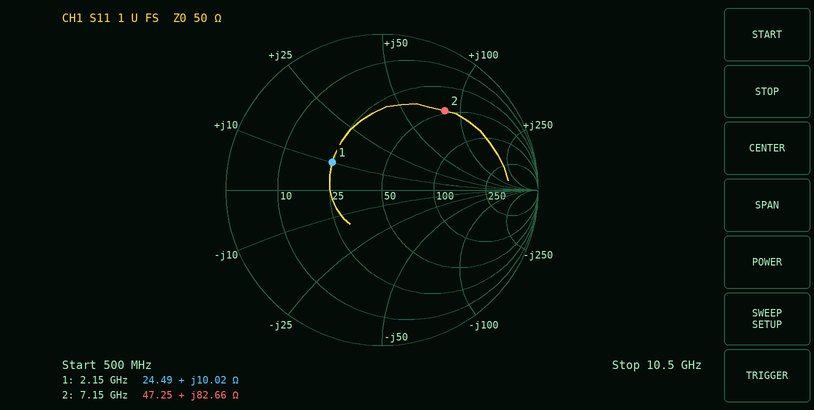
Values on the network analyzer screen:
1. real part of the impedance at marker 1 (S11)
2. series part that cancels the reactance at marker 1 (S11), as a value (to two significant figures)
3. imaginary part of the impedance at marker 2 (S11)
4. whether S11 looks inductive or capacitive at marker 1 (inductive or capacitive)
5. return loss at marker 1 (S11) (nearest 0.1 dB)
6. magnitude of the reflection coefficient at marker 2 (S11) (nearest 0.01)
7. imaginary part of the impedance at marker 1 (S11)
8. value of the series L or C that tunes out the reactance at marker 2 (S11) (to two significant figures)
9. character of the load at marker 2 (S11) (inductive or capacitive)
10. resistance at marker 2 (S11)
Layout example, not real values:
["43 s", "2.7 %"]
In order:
["24.49 Ω", "7.4 pF", "+82.66 Ω", "inductive", "8.8 dB", "0.65", "+10.02 Ω", "270 fF", "inductive", "47.25 Ω"]
